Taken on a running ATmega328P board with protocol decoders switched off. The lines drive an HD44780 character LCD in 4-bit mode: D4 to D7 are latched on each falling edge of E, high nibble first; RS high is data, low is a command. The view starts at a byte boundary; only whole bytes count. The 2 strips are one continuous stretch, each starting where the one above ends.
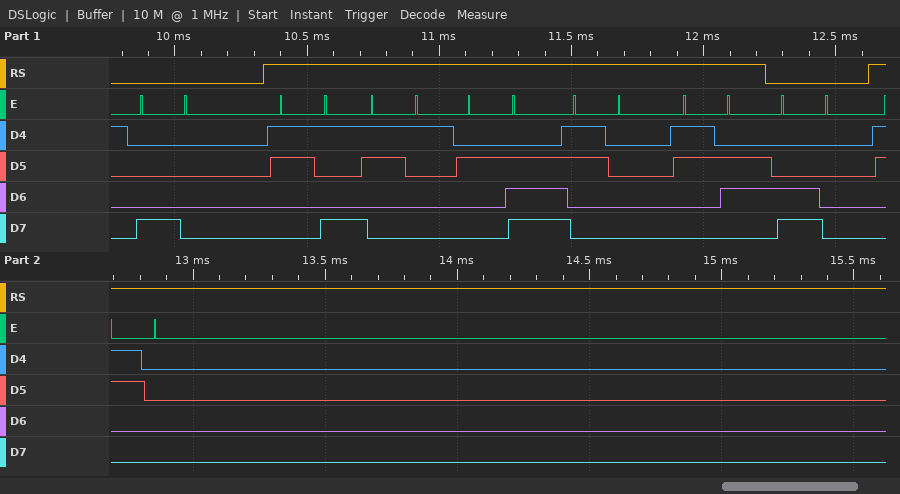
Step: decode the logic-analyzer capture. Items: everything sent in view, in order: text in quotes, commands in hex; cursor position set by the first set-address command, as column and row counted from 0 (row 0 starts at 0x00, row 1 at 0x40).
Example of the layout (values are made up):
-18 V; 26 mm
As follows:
0x80 "91.06" 0xC0 "0"; column 0, row 0
